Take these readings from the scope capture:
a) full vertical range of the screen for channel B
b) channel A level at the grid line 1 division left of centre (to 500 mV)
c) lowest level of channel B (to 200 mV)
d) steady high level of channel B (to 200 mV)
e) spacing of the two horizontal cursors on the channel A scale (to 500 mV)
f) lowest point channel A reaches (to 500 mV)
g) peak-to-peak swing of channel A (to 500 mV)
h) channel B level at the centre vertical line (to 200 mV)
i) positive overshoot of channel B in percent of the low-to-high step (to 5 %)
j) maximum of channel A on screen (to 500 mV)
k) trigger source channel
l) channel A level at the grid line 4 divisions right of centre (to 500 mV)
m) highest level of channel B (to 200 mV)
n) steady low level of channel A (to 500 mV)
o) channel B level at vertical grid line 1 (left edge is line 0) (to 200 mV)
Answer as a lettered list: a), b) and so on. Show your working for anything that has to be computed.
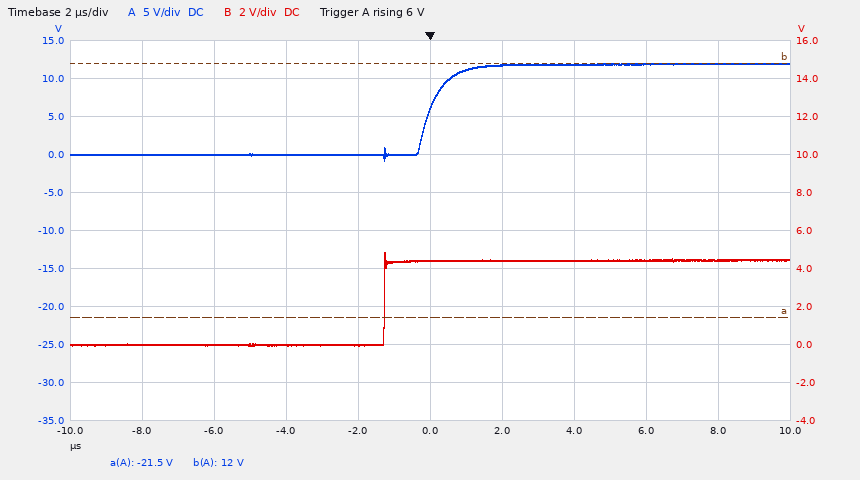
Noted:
a) 20 V
b) 0.0 V
c) 0.0 V
d) 4.4 V
e) 33.5 V
f) -1.0 V
g) 12.0 V − (-1.0 V) = 13.0 V
h) 4.4 V
i) 10 %
j) 12.0 V
k) channel A
l) 12.0 V
m) 4.8 V
n) 0.0 V
o) 0.0 V
